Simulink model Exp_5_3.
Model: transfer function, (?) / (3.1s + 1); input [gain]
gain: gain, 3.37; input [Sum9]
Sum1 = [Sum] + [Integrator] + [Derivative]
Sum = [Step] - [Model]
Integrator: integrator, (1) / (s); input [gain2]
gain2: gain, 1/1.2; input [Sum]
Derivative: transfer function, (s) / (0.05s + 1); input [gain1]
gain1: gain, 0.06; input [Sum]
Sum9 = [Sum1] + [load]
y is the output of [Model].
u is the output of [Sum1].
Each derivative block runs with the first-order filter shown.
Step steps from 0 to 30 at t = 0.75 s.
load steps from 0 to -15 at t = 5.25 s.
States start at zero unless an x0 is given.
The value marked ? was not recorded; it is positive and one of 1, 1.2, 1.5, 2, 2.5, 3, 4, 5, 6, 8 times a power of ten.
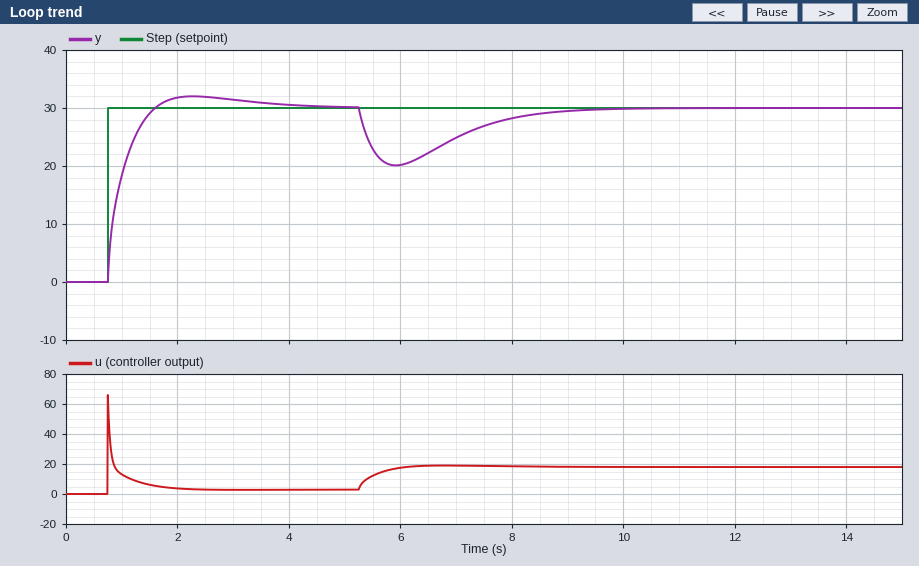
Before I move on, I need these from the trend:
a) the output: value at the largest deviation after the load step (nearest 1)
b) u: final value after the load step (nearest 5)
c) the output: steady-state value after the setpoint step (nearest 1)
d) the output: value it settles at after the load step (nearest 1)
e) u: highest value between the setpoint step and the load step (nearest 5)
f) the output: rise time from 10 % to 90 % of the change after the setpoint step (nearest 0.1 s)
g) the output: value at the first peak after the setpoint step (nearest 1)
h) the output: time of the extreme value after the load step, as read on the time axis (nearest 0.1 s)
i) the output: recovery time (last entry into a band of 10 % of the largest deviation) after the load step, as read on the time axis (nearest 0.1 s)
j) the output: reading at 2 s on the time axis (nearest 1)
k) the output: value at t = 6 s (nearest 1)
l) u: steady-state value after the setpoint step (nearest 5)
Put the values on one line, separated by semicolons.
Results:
20; 20; 30; 30; 65; 0.6 s; 32; 5.9 s; 8.5 s; 32; 20; 5
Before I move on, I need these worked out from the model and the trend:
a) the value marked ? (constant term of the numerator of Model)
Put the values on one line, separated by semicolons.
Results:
3
